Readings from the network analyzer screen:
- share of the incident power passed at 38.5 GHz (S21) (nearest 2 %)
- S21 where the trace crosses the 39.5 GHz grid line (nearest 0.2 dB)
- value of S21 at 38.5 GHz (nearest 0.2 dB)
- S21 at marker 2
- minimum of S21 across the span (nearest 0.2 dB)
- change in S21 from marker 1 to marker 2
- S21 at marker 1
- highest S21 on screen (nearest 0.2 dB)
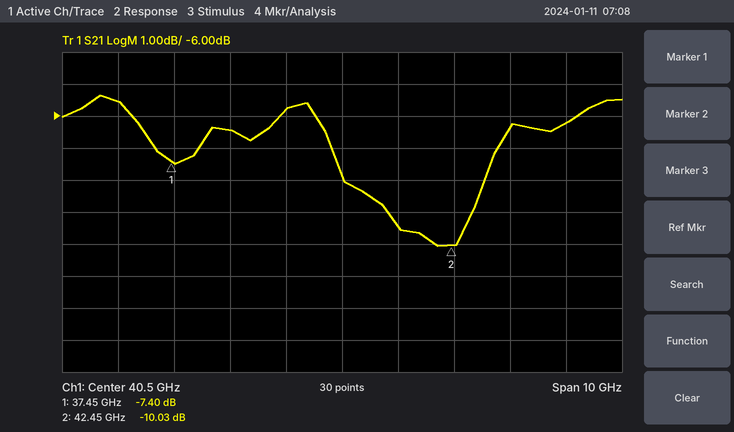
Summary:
22 %
-5.8 dB
-6.4 dB
-10.03 dB
-10.0 dB
-2.63 dB
-7.40 dB
-5.4 dB
